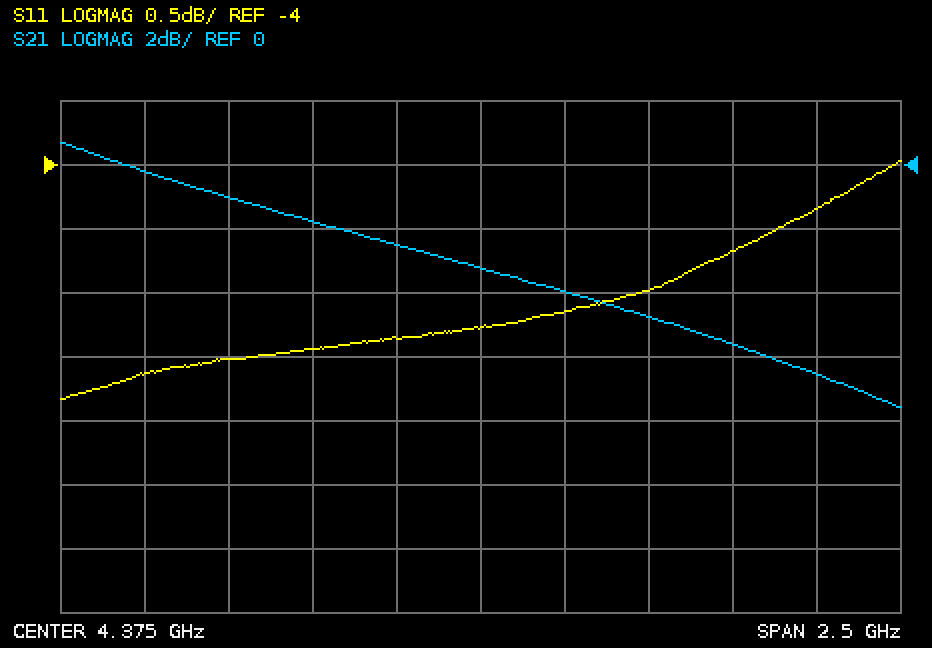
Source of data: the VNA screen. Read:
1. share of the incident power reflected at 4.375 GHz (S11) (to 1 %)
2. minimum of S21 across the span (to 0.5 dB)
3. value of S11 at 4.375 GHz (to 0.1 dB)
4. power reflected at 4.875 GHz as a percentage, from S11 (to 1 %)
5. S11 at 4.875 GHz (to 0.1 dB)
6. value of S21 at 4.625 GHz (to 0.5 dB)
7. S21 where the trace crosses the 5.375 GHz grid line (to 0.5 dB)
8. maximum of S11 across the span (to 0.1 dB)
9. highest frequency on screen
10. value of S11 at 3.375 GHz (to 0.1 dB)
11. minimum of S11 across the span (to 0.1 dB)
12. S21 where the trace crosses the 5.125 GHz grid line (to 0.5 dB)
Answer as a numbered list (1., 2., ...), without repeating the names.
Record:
1. 30 %
2. -7.5 dB
3. -5.3 dB
4. 32 %
5. -5.0 dB
6. -4.0 dB
7. -6.5 dB
8. -4.0 dB
9. 5.625 GHz
10. -5.6 dB
11. -5.8 dB
12. -5.5 dB
